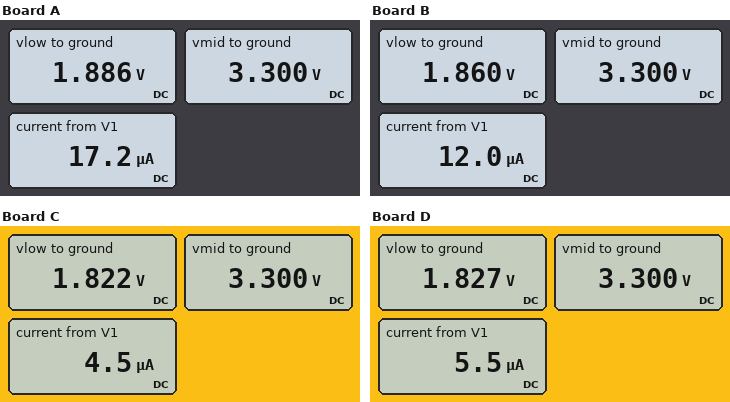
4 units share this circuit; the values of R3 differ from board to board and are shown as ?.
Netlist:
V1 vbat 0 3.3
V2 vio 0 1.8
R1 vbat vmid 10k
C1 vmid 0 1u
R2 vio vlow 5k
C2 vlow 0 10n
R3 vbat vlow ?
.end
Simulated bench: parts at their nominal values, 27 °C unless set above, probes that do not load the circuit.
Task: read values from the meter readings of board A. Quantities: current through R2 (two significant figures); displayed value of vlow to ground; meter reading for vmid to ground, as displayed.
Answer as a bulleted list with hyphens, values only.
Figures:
- 17 µA
- 1.886 V
- 3.300 V
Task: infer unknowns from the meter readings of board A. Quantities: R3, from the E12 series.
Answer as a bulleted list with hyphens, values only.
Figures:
- 82 kΩ
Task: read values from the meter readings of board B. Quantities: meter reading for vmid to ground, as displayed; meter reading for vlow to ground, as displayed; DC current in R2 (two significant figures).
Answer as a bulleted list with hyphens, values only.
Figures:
- 3.300 V
- 1.860 V
- 12 µA
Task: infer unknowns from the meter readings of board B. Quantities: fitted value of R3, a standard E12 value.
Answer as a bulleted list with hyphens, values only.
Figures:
- 120 kΩ
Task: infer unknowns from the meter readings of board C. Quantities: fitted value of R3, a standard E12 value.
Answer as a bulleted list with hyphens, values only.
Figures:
- 330 kΩ
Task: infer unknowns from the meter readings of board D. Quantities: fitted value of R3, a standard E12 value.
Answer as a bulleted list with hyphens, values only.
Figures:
- 270 kΩ
